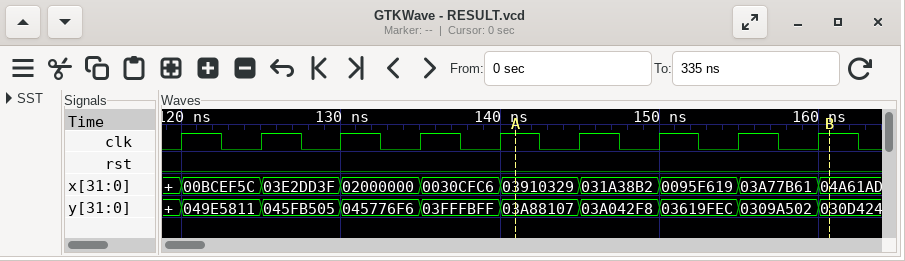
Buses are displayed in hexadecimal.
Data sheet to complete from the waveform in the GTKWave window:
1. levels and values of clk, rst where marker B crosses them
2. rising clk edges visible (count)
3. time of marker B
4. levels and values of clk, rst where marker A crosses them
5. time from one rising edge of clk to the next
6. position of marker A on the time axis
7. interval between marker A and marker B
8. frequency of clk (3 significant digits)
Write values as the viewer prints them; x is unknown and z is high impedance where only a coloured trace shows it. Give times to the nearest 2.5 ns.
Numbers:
clk=1, rst=0
9
160 ns
clk=1, rst=0
5 ns
140 ns
20 ns
200 MHz
